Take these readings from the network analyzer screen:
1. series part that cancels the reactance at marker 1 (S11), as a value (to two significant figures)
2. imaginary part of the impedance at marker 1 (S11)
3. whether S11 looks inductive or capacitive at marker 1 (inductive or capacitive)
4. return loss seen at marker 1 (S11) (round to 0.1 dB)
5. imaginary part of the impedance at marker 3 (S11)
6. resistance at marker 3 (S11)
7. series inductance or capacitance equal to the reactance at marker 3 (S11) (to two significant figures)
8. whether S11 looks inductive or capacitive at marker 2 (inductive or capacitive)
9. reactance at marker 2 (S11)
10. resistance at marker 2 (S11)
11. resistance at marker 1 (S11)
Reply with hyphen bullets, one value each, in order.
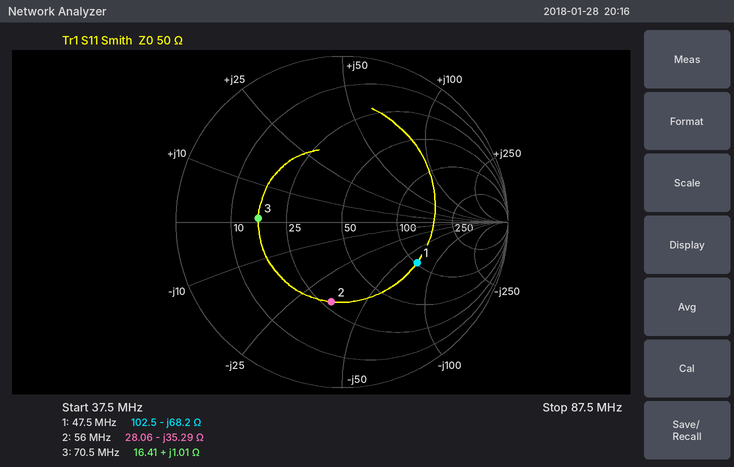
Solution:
- 230 nH
- -68.2 Ω
- capacitive
- 5.8 dB
- +1.01 Ω
- 16.41 Ω
- 2.3 nH
- capacitive
- -35.29 Ω
- 28.06 Ω
- 102.5 Ω
